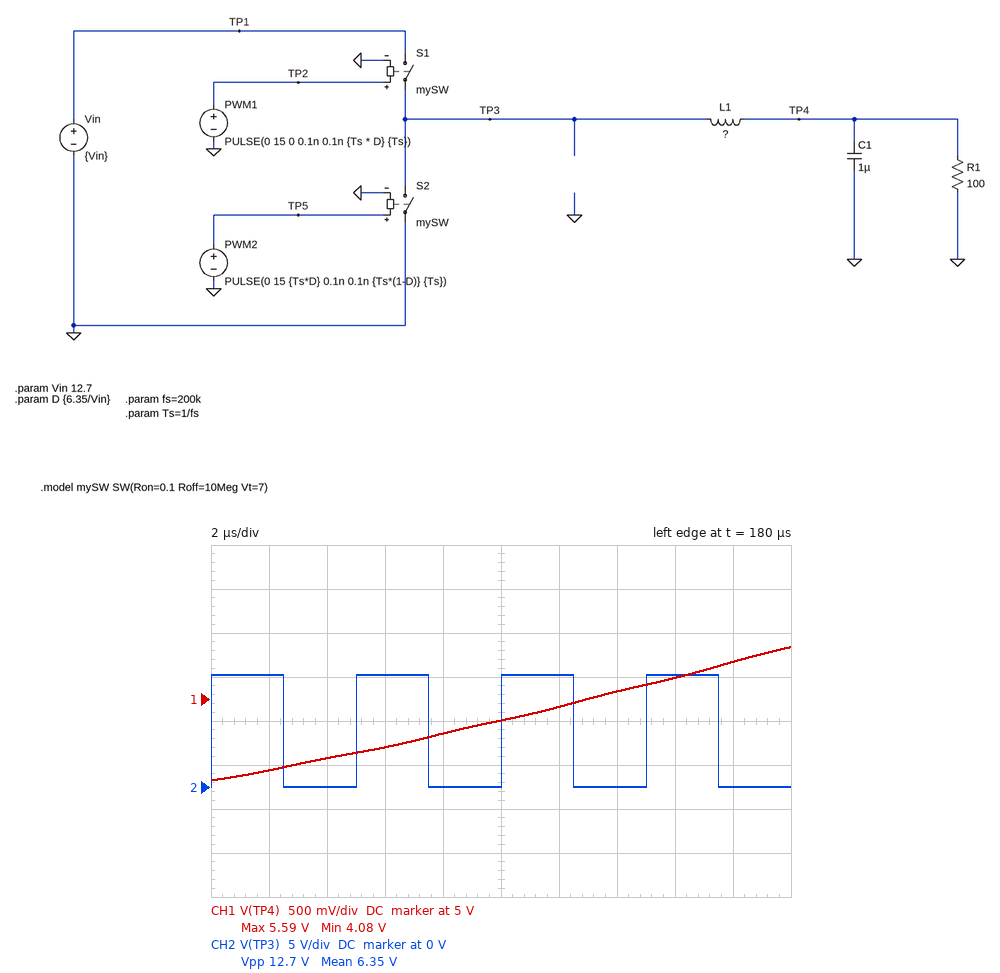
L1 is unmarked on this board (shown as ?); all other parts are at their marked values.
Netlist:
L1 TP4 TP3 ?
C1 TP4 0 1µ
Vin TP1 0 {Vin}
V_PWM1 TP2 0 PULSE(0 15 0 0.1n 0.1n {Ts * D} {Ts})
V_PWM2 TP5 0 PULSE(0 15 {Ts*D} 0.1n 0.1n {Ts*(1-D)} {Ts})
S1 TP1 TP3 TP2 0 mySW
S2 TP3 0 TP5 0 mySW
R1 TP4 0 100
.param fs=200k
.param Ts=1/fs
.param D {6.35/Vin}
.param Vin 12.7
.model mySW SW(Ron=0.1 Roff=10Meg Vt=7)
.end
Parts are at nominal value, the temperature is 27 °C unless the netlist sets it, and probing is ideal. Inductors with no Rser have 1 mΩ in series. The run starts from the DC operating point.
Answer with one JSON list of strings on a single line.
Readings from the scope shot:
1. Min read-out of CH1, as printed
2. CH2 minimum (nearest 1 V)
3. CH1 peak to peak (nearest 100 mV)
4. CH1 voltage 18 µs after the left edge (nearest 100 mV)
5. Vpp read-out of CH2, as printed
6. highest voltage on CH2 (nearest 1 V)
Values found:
["4.08 V", "0 V", "1.5 V", "5.4 V", "12.7 V", "13 V"]
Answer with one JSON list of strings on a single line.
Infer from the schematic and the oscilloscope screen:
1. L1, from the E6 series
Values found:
["680 µH"]
